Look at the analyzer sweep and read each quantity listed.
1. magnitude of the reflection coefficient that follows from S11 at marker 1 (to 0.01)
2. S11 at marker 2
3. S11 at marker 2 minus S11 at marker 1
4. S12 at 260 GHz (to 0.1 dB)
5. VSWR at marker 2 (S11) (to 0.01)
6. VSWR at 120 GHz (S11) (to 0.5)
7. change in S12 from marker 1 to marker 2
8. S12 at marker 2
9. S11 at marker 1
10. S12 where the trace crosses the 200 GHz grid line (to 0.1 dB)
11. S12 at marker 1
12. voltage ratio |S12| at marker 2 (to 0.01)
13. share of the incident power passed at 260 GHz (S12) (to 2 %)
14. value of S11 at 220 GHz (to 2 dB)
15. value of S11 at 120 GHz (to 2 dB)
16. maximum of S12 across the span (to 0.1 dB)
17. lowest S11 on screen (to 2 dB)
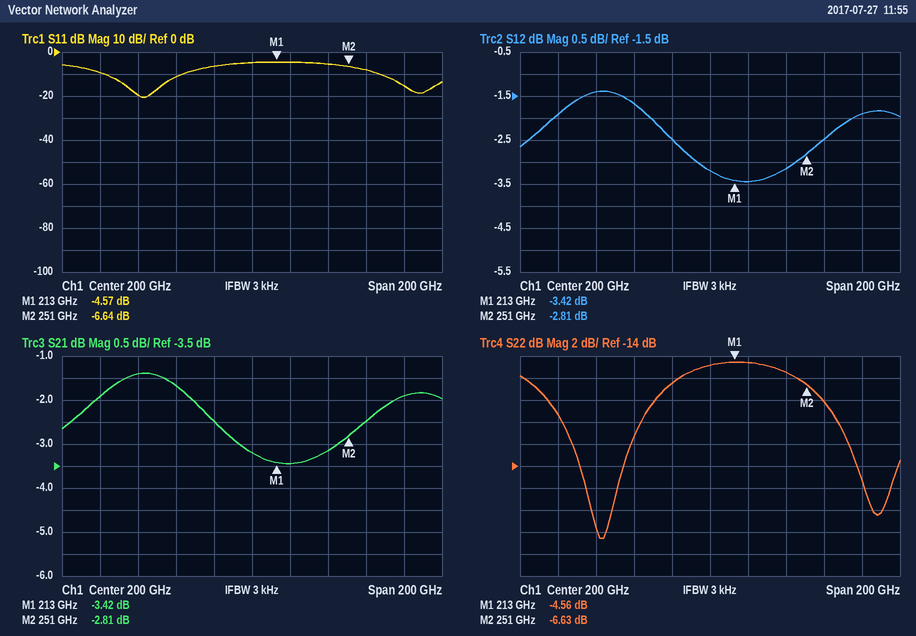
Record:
0.59
-6.64 dB
-2.07 dB
-2.5 dB
2.74
2.0
0.61 dB
-2.81 dB
-4.57 dB
-3.2 dB
-3.42 dB
0.72
56 %
-4 dB
-10 dB
-1.4 dB
-20 dB
